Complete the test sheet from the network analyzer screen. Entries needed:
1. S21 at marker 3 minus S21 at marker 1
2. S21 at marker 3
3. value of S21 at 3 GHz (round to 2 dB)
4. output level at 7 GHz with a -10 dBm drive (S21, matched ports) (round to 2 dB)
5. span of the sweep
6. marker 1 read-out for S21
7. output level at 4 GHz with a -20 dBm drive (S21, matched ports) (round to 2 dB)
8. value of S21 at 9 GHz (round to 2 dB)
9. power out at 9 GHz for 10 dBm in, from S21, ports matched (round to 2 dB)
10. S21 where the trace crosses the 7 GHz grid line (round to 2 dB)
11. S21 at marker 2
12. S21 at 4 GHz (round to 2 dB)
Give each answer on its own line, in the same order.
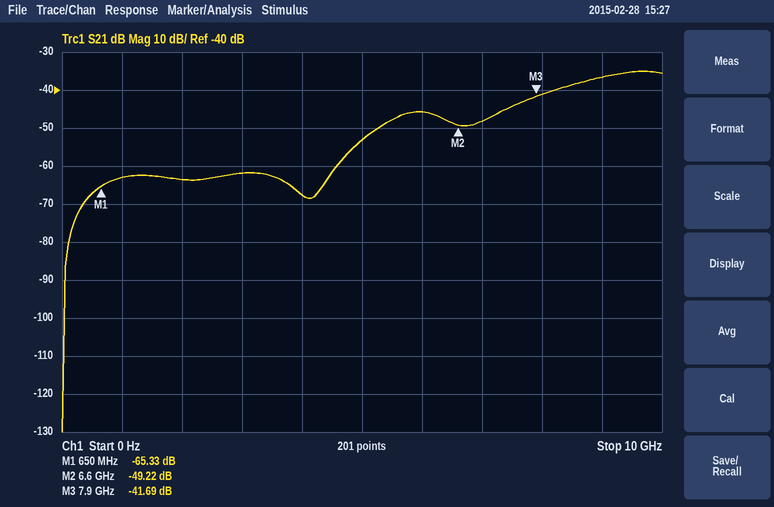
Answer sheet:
23.64 dB
-41.69 dB
-62 dB
-58 dBm
10 GHz
-65.33 dB
-88 dBm
-36 dB
-26 dBm
-48 dB
-49.22 dB
-68 dB
